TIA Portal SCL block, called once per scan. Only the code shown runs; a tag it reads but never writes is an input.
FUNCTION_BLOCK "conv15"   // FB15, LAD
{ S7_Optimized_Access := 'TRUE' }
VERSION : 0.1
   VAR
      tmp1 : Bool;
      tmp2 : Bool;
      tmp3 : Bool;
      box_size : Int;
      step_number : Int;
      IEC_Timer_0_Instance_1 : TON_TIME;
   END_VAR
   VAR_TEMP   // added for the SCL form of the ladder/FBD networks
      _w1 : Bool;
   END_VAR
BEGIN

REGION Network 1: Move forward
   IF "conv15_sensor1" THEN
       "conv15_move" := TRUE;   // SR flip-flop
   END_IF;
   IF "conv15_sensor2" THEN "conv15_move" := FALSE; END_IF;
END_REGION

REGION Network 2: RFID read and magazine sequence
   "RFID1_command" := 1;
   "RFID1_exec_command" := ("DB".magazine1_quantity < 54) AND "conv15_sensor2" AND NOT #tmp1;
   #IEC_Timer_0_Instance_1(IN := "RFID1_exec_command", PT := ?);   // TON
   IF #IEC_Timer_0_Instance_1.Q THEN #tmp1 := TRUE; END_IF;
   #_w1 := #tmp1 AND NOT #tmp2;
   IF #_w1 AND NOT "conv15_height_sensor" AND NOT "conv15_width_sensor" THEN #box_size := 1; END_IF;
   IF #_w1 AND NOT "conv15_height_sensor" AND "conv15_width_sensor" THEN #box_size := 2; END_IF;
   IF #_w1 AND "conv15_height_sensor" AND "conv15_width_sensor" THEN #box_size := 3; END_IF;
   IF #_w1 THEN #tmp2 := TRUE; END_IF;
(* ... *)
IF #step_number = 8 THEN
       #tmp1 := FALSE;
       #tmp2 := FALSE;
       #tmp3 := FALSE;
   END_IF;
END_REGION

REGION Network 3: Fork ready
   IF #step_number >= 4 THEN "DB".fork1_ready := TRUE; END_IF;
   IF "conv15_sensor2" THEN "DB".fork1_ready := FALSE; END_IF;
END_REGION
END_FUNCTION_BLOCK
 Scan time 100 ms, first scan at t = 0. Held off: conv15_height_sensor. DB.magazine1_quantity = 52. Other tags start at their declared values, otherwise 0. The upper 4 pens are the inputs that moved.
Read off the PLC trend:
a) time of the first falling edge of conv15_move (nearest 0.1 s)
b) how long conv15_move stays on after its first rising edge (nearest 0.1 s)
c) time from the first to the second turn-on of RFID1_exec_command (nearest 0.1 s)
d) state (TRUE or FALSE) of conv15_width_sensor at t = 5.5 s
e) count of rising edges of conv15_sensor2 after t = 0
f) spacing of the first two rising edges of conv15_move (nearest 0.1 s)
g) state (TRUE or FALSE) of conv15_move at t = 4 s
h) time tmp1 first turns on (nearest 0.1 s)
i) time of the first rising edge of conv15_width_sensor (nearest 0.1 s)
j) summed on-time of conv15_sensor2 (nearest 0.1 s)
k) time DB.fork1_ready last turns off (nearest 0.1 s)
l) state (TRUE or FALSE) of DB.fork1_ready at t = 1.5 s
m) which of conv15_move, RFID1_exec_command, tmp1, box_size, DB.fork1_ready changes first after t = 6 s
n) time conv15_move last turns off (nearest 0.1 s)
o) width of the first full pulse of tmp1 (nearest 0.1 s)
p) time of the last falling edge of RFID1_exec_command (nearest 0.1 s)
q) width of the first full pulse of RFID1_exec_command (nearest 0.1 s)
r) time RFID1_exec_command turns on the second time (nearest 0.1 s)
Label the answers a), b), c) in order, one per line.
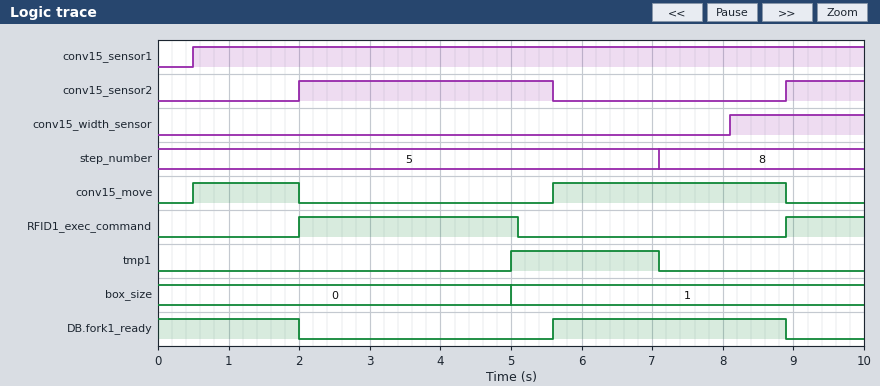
a) 2.0 s
b) 1.5 s
c) 6.9 s
d) FALSE
e) 2
f) 5.1 s
g) FALSE
h) 5.0 s
i) 8.1 s
j) 4.7 s
k) 8.9 s
l) TRUE
m) tmp1
n) 8.9 s
o) 2.1 s
p) 5.1 s
q) 3.1 s
r) 8.9 s
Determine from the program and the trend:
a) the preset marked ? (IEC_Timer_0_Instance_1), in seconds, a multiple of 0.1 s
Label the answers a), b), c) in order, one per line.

a) 3.0 s
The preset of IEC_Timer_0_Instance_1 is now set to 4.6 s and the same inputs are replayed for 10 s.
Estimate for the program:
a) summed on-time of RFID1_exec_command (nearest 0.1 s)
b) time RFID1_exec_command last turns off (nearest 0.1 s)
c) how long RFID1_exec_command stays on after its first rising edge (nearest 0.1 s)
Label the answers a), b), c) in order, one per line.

a) 4.7 s
b) 5.6 s
c) 3.6 s
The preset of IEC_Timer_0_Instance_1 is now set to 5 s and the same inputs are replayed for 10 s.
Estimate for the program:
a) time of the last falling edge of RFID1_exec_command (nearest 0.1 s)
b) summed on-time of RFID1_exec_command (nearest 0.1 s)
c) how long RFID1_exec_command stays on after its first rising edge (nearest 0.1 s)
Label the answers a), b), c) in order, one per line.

a) 5.6 s
b) 4.7 s
c) 3.6 s
